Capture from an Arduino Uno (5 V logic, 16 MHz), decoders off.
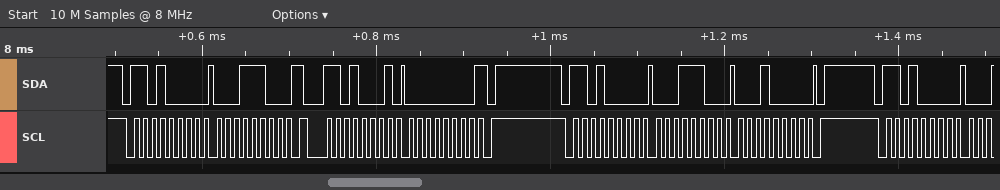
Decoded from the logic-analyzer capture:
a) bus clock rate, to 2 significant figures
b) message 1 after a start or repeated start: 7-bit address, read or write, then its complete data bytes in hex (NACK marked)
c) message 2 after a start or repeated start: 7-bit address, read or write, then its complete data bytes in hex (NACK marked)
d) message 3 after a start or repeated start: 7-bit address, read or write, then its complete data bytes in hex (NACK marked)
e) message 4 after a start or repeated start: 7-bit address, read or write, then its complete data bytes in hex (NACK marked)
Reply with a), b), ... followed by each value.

a) 100 kHz
b) 0x68 write: 1C
c) 0x68 read: 00 NACK
d) 0x68 write: 1C 10
e) 0x68 write
